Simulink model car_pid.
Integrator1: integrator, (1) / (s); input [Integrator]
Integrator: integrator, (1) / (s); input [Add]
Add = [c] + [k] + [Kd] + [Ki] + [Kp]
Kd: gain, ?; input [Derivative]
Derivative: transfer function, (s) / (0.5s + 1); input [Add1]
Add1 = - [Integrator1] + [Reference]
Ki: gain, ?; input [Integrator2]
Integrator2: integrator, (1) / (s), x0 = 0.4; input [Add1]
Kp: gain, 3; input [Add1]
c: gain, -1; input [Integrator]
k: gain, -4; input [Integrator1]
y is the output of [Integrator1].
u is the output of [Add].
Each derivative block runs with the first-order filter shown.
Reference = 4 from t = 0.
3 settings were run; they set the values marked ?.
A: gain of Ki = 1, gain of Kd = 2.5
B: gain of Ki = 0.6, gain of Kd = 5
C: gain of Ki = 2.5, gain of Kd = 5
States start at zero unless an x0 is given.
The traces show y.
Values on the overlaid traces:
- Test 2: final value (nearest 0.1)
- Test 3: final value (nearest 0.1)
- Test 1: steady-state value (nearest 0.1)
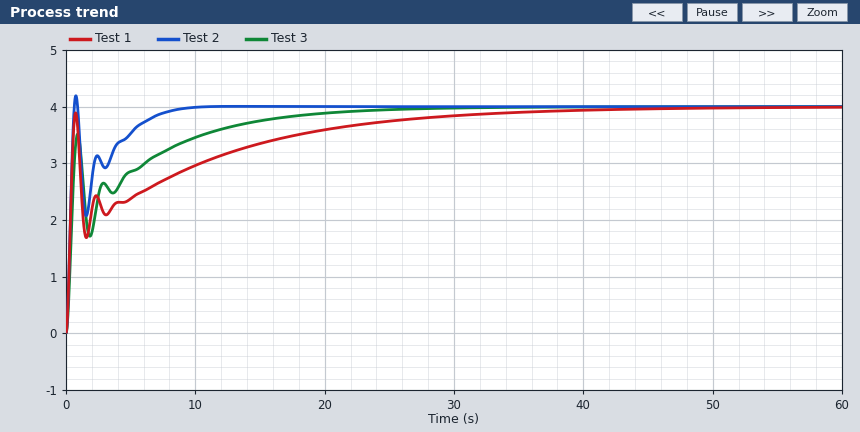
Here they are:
4.0
4.0
4.0
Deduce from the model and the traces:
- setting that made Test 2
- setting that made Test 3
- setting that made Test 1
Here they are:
C
A
B
